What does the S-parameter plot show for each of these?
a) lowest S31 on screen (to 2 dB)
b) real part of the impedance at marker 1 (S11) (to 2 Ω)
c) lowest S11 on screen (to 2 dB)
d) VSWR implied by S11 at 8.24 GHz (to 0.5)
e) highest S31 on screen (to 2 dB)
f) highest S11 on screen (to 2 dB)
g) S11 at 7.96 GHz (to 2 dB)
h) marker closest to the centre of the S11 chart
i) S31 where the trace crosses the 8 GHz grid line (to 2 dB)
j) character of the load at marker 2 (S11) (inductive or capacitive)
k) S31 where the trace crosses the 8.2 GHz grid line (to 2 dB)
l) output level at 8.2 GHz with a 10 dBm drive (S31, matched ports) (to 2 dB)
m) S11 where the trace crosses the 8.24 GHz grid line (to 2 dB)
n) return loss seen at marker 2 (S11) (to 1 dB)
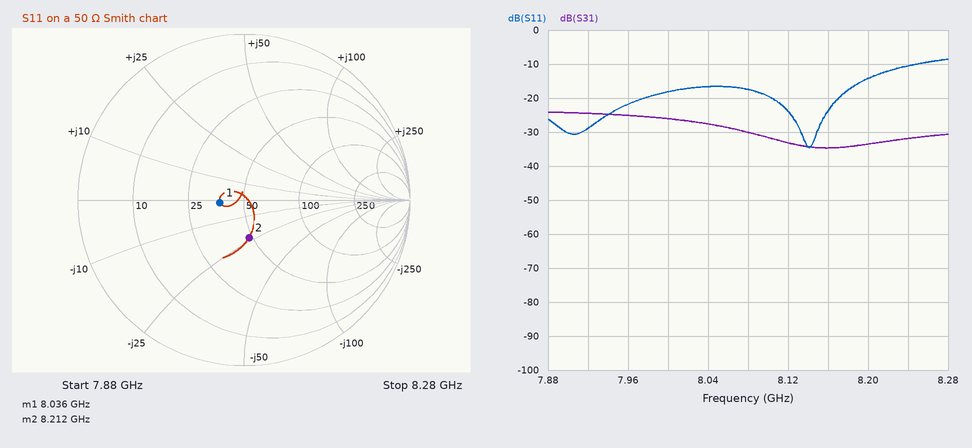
-34 dB
38 Ω
-34 dB
2.0
-24 dB
-8 dB
-22 dB
marker 1
-26 dB
capacitive
-34 dB
-24 dBm
-10 dB
13 dB
